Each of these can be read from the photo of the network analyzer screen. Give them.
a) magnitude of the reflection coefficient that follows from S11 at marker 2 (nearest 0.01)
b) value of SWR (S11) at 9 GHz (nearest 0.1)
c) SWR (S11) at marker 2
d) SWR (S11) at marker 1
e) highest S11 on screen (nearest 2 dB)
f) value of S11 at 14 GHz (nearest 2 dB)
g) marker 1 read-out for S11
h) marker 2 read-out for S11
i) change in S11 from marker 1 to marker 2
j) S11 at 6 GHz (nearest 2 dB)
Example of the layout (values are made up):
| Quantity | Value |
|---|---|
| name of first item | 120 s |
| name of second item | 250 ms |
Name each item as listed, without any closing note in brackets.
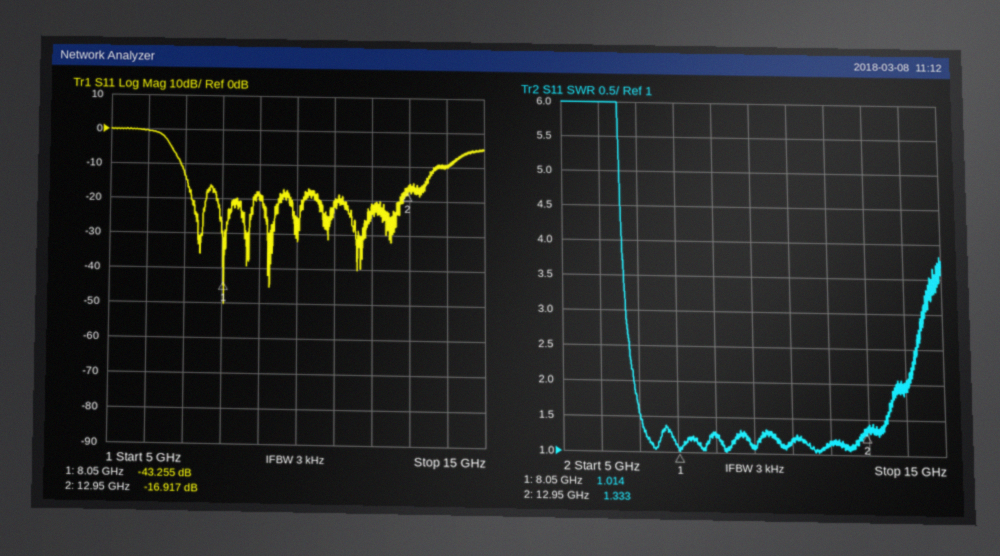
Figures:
| Quantity | Value |
|---|---|
| magnitude of the reflection coefficient that follows from S11 at marker 2 | 0.14 |
| value of SWR (S11) at 9 GHz | 1.2 |
| SWR (S11) at marker 2 | 1.333 |
| SWR (S11) at marker 1 | 1.014 |
| highest S11 on screen | 0 dB |
| value of S11 at 14 GHz | -10 dB |
| marker 1 read-out for S11 | -43.255 dB |
| marker 2 read-out for S11 | -16.917 dB |
| change in S11 from marker 1 to marker 2 | 26.338 dB |
| S11 at 6 GHz | 0 dB |
